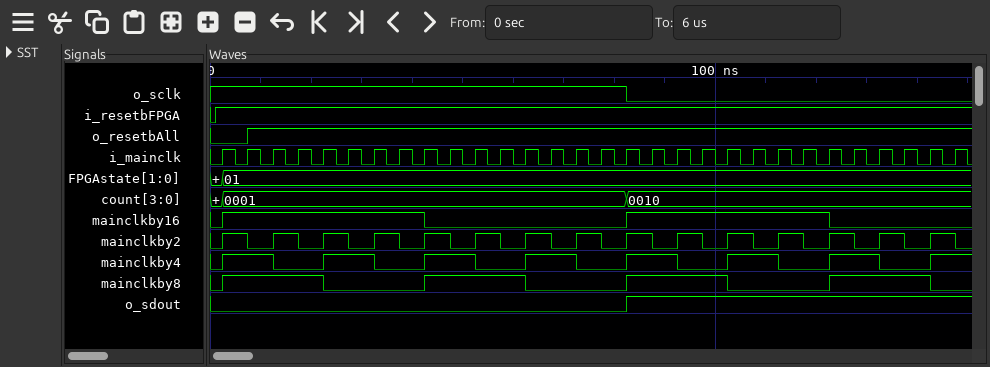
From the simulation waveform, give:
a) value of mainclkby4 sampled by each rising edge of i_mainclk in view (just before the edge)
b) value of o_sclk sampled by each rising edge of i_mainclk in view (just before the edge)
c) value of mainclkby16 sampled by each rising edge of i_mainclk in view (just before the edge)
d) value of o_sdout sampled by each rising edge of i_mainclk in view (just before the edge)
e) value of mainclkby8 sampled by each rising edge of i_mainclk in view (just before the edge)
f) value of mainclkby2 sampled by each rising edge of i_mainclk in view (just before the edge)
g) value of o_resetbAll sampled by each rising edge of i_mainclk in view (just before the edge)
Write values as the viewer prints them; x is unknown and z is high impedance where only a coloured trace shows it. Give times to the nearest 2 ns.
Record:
0 1 1 0 0 1 1 0 0 1 1 0 0 1 1 0 0 1 1 0 0 1 1 0 0 1 1 0 0 1
1 1 1 1 1 1 1 1 1 1 1 1 1 1 1 1 1 0 0 0 0 0 0 0 0 0 0 0 0 0
0 1 1 1 1 1 1 1 1 0 0 0 0 0 0 0 0 1 1 1 1 1 1 1 1 0 0 0 0 0
0 0 0 0 0 0 0 0 0 0 0 0 0 0 0 0 0 1 1 1 1 1 1 1 1 1 1 1 1 1
0 1 1 1 1 0 0 0 0 1 1 1 1 0 0 0 0 1 1 1 1 0 0 0 0 1 1 1 1 0
0 1 0 1 0 1 0 1 0 1 0 1 0 1 0 1 0 1 0 1 0 1 0 1 0 1 0 1 0 1
0 0 1 1 1 1 1 1 1 1 1 1 1 1 1 1 1 1 1 1 1 1 1 1 1 1 1 1 1 1
